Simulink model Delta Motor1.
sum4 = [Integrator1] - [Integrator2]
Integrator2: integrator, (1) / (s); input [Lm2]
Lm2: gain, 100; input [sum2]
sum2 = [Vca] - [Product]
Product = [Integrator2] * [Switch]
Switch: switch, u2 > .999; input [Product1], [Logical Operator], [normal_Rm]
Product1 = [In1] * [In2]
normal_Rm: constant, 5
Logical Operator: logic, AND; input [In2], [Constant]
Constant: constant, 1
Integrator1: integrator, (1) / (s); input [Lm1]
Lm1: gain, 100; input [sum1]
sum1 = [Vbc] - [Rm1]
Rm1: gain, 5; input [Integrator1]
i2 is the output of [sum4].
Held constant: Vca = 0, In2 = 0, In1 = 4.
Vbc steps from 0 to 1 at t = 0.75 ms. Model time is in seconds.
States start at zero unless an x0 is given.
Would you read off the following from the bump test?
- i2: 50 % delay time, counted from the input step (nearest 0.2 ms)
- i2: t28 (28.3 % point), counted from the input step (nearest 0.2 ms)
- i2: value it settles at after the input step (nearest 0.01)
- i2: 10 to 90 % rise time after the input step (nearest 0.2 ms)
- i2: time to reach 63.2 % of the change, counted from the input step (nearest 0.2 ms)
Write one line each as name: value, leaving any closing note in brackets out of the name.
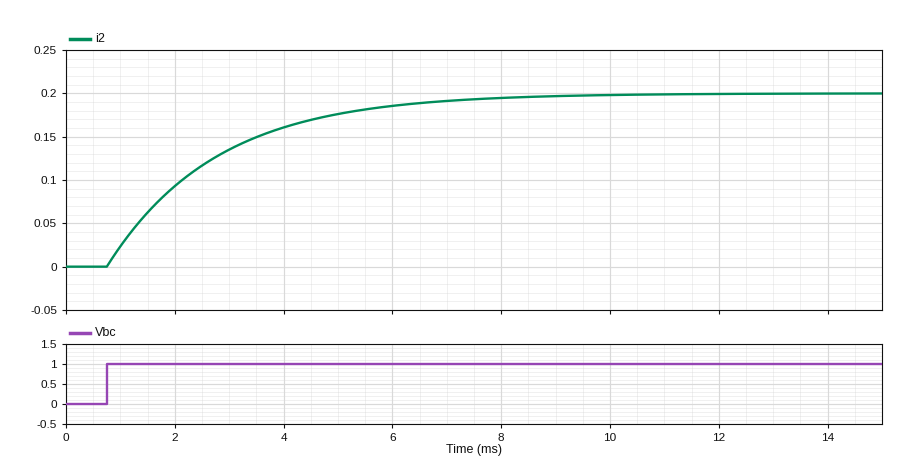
i2: 50 % delay time, counted from the input step: 1.4 ms
i2: t28 (28.3 % point), counted from the input step: 0.6 ms
i2: value it settles at after the input step: 0.20
i2: 10 to 90 % rise time after the input step: 4.4 ms
i2: time to reach 63.2 % of the change, counted from the input step: 2.0 ms
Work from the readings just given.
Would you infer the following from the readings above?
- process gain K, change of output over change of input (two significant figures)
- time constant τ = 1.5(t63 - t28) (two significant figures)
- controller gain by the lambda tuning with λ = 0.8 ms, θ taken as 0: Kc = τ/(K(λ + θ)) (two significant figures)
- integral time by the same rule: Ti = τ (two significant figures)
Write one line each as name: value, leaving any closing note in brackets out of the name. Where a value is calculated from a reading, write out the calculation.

process gain K, change of output over change of input: (0.2 - 0) / 1 = 0.20
time constant τ = 1.5(t63 - t28): 1.5 × (2 - 0.6) = 2.1 ms
controller gain by the lambda tuning with λ = 0.8 ms, θ taken as 0: Kc = τ/(K(λ + θ)): 2.1 / (0.2 × (0.8 + 0)) = 13
integral time by the same rule: Ti = τ: 2.1 ms
